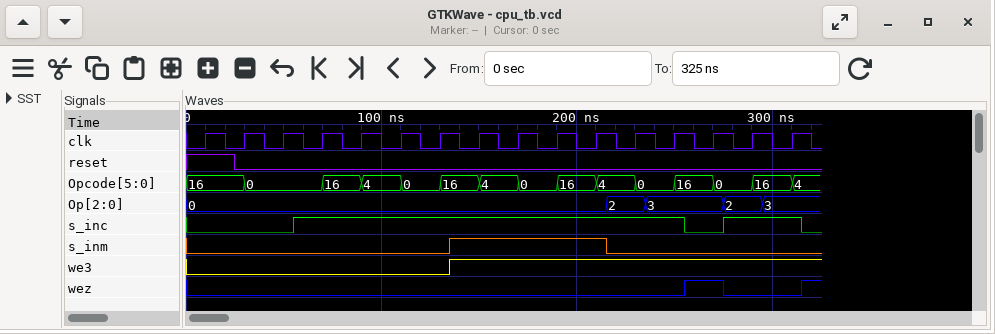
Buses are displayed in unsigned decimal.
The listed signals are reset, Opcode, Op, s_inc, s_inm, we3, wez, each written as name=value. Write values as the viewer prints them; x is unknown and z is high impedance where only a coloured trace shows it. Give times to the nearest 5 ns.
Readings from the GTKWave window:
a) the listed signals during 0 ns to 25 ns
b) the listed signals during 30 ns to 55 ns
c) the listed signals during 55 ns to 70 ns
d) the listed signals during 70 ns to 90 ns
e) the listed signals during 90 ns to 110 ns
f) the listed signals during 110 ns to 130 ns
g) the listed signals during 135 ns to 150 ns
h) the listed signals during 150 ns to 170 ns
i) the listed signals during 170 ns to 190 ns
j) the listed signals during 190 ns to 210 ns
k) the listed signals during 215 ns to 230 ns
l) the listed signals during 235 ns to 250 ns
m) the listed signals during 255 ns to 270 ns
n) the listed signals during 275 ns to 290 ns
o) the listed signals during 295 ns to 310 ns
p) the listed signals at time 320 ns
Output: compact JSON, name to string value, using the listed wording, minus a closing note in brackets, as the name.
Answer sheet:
{"the listed signals during 0 ns to 25 ns": "reset=1, Opcode=16, Op=0, s_inc=0, s_inm=0, we3=0, wez=0", "the listed signals during 30 ns to 55 ns": "reset=0, Opcode=0, Op=0, s_inc=0, s_inm=0, we3=0, wez=0", "the listed signals during 55 ns to 70 ns": "reset=0, Opcode=0, Op=0, s_inc=1, s_inm=0, we3=0, wez=0", "the listed signals during 70 ns to 90 ns": "reset=0, Opcode=16, Op=0, s_inc=1, s_inm=0, we3=0, wez=0", "the listed signals during 90 ns to 110 ns": "reset=0, Opcode=4, Op=0, s_inc=1, s_inm=0, we3=0, wez=0", "the listed signals during 110 ns to 130 ns": "reset=0, Opcode=0, Op=0, s_inc=1, s_inm=0, we3=0, wez=0", "the listed signals during 135 ns to 150 ns": "reset=0, Opcode=16, Op=0, s_inc=1, s_inm=1, we3=1, wez=0", "the listed signals during 150 ns to 170 ns": "reset=0, Opcode=4, Op=0, s_inc=1, s_inm=1, we3=1, wez=0", "the listed signals during 170 ns to 190 ns": "reset=0, Opcode=0, Op=0, s_inc=1, s_inm=1, we3=1, wez=0", "the listed signals during 190 ns to 210 ns": "reset=0, Opcode=16, Op=0, s_inc=1, s_inm=1, we3=1, wez=0", "the listed signals during 215 ns to 230 ns": "reset=0, Opcode=4, Op=2, s_inc=1, s_inm=0, we3=1, wez=0", "the listed signals during 235 ns to 250 ns": "reset=0, Opcode=0, Op=3, s_inc=1, s_inm=0, we3=1, wez=0", "the listed signals during 255 ns to 270 ns": "reset=0, Opcode=16, Op=3, s_inc=0, s_inm=0, we3=1, wez=1", "the listed signals during 275 ns to 290 ns": "reset=0, Opcode=0, Op=2, s_inc=1, s_inm=0, we3=1, wez=0", "the listed signals during 295 ns to 310 ns": "reset=0, Opcode=16, Op=3, s_inc=1, s_inm=0, we3=1, wez=0", "the listed signals at time 320 ns": "reset=0, Opcode=4, Op=3, s_inc=0, s_inm=0, we3=1, wez=1"}
